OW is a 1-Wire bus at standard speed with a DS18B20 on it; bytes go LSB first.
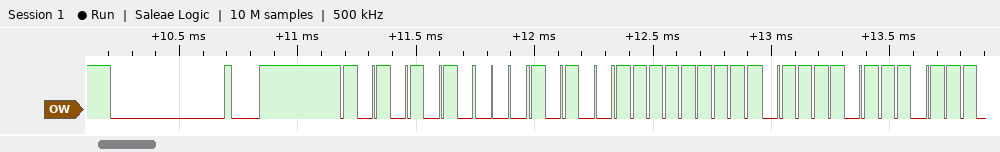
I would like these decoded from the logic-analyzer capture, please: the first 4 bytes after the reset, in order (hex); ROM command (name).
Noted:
55 28 FF BD
Match ROM
